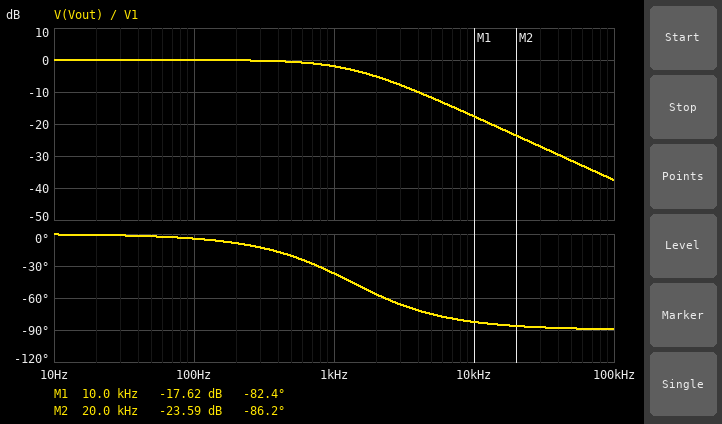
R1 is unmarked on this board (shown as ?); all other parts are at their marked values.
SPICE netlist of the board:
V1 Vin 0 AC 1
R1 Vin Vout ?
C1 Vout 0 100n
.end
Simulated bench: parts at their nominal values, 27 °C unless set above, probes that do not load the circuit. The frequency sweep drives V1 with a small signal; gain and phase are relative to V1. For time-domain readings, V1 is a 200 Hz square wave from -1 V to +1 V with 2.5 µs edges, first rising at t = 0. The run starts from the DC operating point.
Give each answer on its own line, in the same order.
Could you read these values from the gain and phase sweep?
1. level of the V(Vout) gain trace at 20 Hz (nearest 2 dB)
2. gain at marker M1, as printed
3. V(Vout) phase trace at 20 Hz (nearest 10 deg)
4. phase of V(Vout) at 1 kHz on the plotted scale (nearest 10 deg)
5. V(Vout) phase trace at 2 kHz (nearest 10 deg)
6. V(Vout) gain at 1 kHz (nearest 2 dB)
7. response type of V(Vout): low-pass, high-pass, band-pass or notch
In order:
0 dB
-17.62 dB
0 deg
-40 deg
-60 deg
-2 dB
low-pass
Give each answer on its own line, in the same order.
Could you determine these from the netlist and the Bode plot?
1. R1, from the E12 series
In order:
1.2 kΩ
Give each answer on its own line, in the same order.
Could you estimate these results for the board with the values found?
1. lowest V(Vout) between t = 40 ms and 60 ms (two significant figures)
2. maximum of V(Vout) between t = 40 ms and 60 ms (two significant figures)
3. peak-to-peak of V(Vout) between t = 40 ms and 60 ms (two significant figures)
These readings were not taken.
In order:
-1.0 V
1.0 V
2.0 V
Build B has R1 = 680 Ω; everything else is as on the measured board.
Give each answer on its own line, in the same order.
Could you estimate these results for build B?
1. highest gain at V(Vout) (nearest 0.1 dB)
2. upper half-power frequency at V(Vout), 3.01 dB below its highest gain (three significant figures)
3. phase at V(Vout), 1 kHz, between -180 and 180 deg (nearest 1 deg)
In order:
0 dB
2.34 kHz
-23 deg
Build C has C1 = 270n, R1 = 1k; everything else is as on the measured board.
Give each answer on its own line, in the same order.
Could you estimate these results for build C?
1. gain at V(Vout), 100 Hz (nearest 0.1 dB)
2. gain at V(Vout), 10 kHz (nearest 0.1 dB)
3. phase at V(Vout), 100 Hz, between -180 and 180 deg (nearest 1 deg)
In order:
-0.1 dB
-24.6 dB
-10 deg
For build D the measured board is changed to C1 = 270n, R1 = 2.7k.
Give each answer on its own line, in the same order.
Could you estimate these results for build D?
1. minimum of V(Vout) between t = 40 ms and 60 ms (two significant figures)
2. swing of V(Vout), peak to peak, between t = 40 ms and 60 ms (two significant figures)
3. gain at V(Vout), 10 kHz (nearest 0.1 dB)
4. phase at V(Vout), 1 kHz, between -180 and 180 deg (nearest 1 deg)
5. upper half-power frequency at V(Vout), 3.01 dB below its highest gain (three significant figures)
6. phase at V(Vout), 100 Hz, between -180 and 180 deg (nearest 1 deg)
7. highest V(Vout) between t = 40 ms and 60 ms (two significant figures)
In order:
-940 mV
1.9 V
-33.2 dB
-78 deg
218 Hz
-25 deg
940 mV
